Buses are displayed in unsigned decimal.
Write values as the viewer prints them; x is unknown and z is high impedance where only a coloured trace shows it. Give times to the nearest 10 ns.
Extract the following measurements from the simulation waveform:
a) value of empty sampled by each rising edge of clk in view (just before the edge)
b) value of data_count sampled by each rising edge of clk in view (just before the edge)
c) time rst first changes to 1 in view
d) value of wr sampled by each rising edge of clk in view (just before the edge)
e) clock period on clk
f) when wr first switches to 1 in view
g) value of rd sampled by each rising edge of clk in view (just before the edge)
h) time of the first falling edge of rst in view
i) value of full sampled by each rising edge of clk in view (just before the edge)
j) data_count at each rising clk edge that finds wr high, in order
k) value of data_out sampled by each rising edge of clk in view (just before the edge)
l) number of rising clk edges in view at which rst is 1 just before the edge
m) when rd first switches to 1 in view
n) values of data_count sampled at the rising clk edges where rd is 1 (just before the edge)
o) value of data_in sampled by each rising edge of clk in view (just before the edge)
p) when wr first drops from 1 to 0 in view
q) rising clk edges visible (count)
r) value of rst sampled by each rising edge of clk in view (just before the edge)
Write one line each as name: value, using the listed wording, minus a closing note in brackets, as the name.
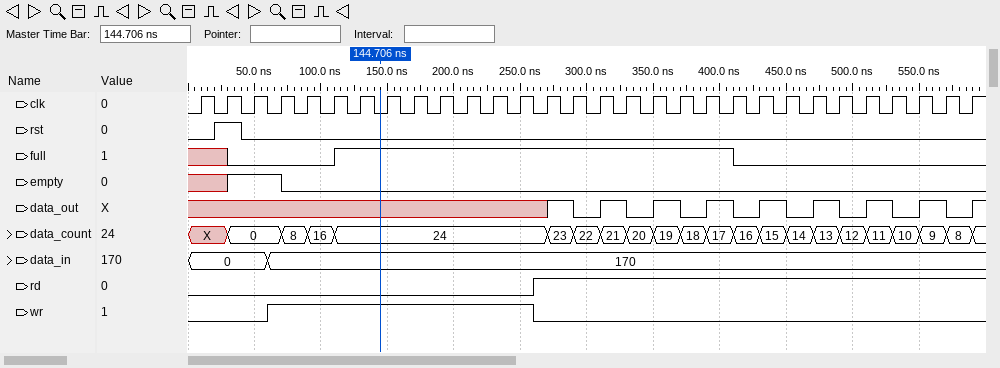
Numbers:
value of empty sampled by each rising edge of clk in view: x x 1 1 0 0 0 0 0 0 0 0 0 0 0 0 0 0 0 0 0 0 0 0 0 0 0 0 0 0
value of data_count sampled by each rising edge of clk in view: X, X, 0, 0, 8, 16, 24, 24, 24, 24, 24, 24, 24, 24, 23, 22, 21, 20, 19, 18, 17, 16, 15, 14, 13, 12, 11, 10, 9, 8
time rst first changes to 1 in view: 20 ns
value of wr sampled by each rising edge of clk in view: 0 0 0 1 1 1 1 1 1 1 1 1 1 0 0 0 0 0 0 0 0 0 0 0 0 0 0 0 0 0
clock period on clk: 20 ns
when wr first switches to 1 in view: 60 ns
value of rd sampled by each rising edge of clk in view: 0 0 0 0 0 0 0 0 0 0 0 0 0 1 1 1 1 1 1 1 1 1 1 1 1 1 1 1 1 1
time of the first falling edge of rst in view: 40 ns
value of full sampled by each rising edge of clk in view: x x 0 0 0 0 1 1 1 1 1 1 1 1 1 1 1 1 1 1 1 0 0 0 0 0 0 0 0 0
data_count at each rising clk edge that finds wr high, in order: 0, 8, 16, 24, 24, 24, 24, 24, 24, 24
value of data_out sampled by each rising edge of clk in view: x x x x x x x x x x x x x x 1 0 1 0 1 0 1 0 1 0 1 0 1 0 1 0
number of rising clk edges in view at which rst is 1 just before the edge: 1
when rd first switches to 1 in view: 260 ns
values of data_count sampled at the rising clk edges where rd is 1: 24, 23, 22, 21, 20, 19, 18, 17, 16, 15, 14, 13, 12, 11, 10, 9, 8
value of data_in sampled by each rising edge of clk in view: 0, 0, 0, 170, 170, 170, 170, 170, 170, 170, 170, 170, 170, 170, 170, 170, 170, 170, 170, 170, 170, 170, 170, 170, 170, 170, 170, 170, 170, 170
when wr first drops from 1 to 0 in view: 260 ns
rising clk edges visible: 30
value of rst sampled by each rising edge of clk in view: 0 1 0 0 0 0 0 0 0 0 0 0 0 0 0 0 0 0 0 0 0 0 0 0 0 0 0 0 0 0
